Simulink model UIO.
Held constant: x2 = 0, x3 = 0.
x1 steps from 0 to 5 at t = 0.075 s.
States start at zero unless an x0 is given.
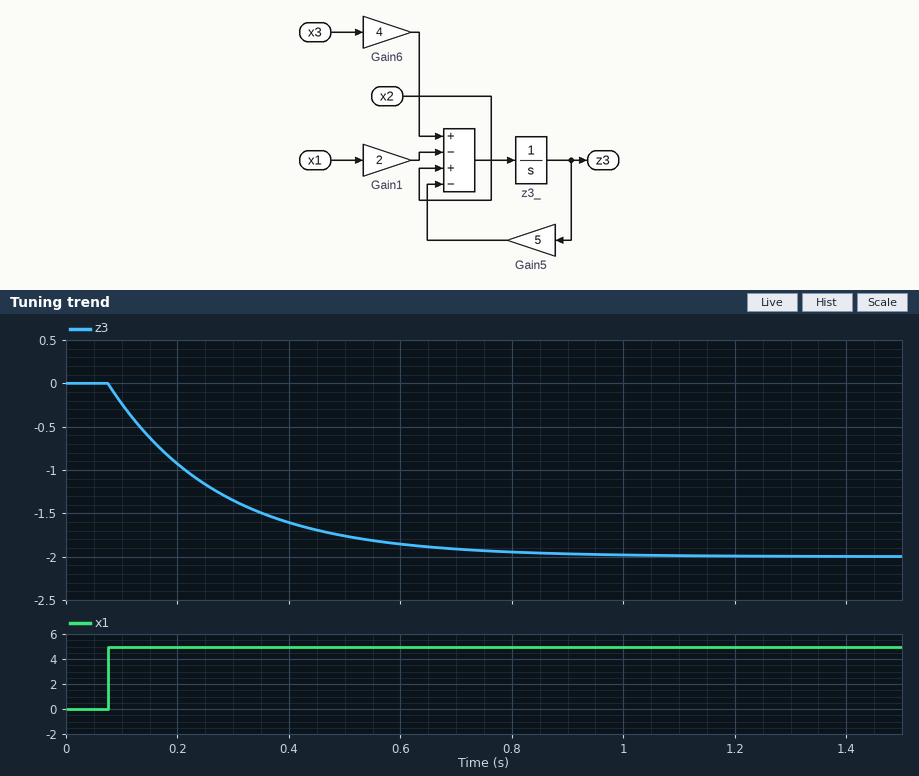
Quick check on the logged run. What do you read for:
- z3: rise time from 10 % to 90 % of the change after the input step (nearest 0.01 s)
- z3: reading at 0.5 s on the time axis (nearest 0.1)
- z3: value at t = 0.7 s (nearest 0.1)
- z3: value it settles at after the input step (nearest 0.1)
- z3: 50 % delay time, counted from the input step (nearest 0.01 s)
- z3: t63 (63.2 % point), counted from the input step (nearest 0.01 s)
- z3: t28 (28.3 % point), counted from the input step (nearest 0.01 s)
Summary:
0.44 s
-1.8
-1.9
-2.0
0.14 s
0.20 s
0.07 s
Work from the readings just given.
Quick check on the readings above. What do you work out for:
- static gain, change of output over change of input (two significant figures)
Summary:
-0.40
